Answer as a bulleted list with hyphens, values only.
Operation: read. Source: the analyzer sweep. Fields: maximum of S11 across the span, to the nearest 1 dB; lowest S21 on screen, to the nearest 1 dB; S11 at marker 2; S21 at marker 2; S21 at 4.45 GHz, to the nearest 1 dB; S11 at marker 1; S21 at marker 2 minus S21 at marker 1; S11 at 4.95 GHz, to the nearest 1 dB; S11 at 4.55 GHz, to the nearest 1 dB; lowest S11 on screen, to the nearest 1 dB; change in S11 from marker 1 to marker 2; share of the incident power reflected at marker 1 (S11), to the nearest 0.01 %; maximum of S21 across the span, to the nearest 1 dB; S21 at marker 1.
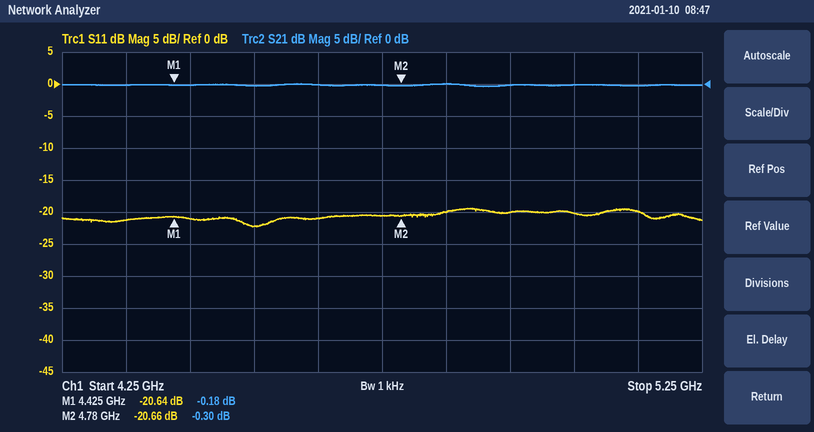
- -19 dB
- 0 dB
- -20.66 dB
- -0.30 dB
- 0 dB
- -20.64 dB
- -0.12 dB
- -20 dB
- -22 dB
- -22 dB
- -0.02 dB
- 0.86 %
- 0 dB
- -0.18 dB
